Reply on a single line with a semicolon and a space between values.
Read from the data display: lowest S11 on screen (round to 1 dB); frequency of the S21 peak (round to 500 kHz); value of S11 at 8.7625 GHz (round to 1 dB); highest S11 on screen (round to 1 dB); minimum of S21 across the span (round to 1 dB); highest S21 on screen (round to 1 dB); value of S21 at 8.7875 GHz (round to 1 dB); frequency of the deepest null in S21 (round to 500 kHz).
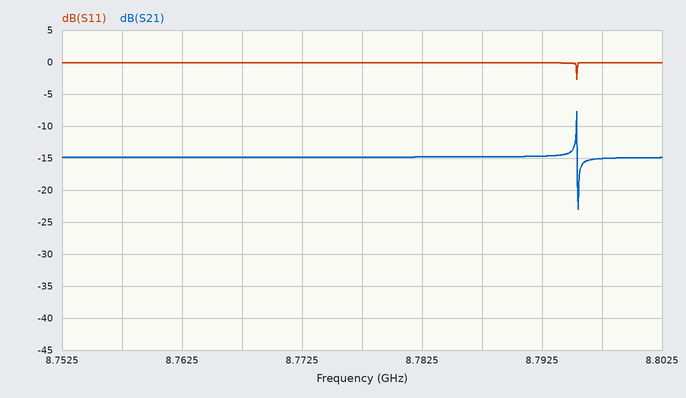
-3 dB; 8.7955 GHz; 0 dB; 0 dB; -23 dB; -8 dB; -15 dB; 8.7955 GHz
